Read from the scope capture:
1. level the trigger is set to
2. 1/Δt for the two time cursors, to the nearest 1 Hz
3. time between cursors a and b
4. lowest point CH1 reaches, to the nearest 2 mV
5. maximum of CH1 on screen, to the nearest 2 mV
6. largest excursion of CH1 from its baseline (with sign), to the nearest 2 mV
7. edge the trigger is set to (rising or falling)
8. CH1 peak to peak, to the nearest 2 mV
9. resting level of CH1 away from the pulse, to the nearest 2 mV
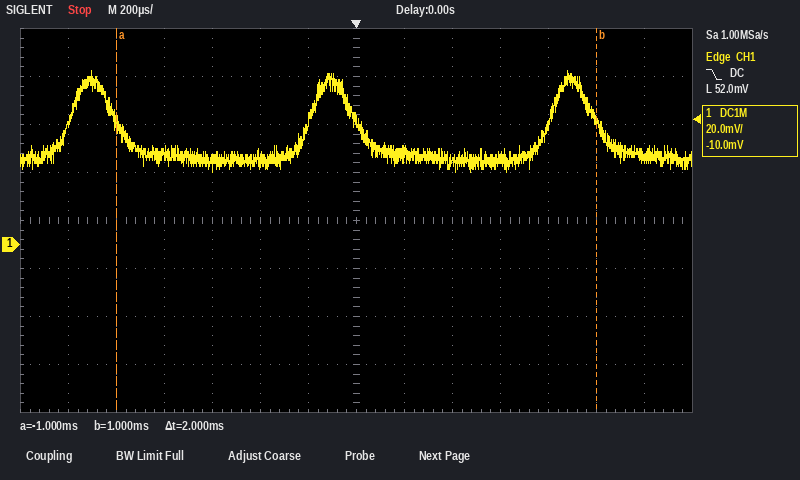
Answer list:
52.0 mV
500 Hz
2 ms
30 mV
72 mV
+36 mV
falling
42 mV
36 mV
